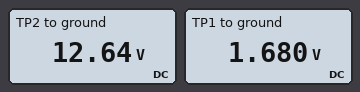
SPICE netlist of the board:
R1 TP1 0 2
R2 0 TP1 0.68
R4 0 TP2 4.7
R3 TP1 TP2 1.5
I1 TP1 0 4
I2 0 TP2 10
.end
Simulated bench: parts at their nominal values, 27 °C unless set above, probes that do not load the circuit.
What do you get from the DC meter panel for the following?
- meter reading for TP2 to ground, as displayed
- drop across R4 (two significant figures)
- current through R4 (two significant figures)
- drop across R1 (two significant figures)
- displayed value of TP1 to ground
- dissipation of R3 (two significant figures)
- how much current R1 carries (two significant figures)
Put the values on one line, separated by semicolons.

12.64 V; 13 V; 2.7 A; 1.7 V; 1.680 V; 80 W; 840 mA
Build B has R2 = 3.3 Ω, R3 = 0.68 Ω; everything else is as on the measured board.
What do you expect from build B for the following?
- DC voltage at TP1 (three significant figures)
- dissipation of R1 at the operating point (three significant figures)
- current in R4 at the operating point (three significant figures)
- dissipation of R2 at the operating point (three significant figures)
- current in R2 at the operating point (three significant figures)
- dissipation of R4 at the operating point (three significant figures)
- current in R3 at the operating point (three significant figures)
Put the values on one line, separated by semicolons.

4.79 V; 11.5 W; 2.15 A; 6.95 W; 1.45 A; 21.8 W; 7.85 A
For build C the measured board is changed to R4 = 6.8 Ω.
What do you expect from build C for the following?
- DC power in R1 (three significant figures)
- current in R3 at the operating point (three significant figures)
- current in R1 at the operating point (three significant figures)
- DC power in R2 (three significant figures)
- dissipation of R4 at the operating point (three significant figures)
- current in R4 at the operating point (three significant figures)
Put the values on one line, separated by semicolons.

2.01 W; 7.95 A; 1.00 A; 5.91 W; 28.5 W; 2.05 A
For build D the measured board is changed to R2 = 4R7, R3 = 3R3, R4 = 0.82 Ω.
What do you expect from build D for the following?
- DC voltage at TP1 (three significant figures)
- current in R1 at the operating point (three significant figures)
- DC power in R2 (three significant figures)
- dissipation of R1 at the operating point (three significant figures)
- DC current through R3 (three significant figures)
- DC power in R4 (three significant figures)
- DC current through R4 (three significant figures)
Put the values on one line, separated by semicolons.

-2.10 V; 1.05 A; 941 mW; 2.21 W; 2.50 A; 46.1 W; 7.50 A
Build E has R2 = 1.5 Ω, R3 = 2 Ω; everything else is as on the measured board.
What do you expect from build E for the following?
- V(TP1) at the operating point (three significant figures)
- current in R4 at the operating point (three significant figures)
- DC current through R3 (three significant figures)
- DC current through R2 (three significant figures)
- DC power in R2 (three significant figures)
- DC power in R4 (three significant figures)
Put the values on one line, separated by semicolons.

2.29 V; 3.33 A; 6.67 A; 1.53 A; 3.50 W; 52.0 W
